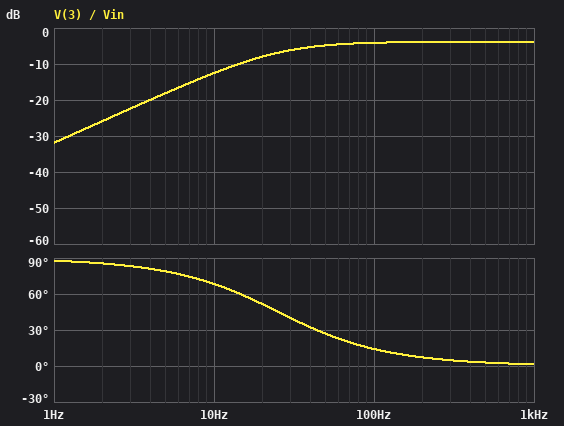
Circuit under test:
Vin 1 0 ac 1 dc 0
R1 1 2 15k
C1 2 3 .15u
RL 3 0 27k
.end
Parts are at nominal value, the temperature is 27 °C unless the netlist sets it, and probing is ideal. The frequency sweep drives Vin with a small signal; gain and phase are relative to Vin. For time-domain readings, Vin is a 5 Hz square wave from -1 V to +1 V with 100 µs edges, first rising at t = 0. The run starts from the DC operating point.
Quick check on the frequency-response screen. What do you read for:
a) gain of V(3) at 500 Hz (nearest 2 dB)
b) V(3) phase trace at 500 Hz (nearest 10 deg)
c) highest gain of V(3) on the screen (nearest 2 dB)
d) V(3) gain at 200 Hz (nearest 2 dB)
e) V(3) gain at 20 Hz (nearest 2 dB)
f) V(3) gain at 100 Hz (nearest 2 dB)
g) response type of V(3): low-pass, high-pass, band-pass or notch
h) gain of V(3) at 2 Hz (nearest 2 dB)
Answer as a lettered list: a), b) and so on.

a) -4 dB
b) 0 deg
c) -4 dB
d) -4 dB
e) -8 dB
f) -4 dB
g) high-pass
h) -26 dB
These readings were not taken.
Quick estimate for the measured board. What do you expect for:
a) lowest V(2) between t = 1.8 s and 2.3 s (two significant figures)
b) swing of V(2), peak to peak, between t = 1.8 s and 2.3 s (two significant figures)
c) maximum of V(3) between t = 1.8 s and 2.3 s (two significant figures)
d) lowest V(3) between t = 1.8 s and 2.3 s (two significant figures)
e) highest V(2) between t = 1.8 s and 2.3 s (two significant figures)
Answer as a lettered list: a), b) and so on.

a) -1.0 V
b) 2.0 V
c) 1.3 V
d) -1.3 V
e) 1.0 V
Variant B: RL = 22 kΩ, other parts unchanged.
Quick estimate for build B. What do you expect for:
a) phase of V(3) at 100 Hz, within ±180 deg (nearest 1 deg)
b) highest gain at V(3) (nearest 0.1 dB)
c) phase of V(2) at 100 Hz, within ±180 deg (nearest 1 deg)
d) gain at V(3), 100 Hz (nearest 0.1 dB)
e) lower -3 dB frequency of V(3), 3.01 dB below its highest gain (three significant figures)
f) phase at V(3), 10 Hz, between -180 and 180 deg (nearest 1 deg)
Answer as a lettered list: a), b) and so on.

a) 16 deg
b) -4.5 dB
c) -10 deg
d) -4.9 dB
e) 28.7 Hz
f) 71 deg
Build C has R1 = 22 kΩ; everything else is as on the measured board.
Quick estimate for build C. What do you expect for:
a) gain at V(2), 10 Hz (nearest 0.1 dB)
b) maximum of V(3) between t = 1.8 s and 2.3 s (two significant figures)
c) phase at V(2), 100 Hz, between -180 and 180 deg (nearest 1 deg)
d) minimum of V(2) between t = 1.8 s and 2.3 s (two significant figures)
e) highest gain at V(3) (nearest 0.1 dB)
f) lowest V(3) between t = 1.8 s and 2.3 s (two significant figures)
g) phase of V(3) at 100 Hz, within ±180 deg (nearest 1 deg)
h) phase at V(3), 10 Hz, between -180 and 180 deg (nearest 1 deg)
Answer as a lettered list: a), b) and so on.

a) -0.6 dB
b) 1.1 V
c) -9 deg
d) -1.0 V
e) -5.2 dB
f) -1.1 V
g) 12 deg
h) 65 deg
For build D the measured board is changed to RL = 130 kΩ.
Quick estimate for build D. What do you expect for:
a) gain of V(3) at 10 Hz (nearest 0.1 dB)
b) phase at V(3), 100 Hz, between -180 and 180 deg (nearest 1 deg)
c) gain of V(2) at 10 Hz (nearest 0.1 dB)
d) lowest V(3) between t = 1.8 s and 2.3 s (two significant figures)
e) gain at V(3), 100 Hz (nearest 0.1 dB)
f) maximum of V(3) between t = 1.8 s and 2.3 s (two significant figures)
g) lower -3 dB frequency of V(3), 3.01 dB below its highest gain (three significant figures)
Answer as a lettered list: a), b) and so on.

a) -2.8 dB
b) 4 deg
c) -0.6 dB
d) -1.8 V
e) -1.0 dB
f) 1.8 V
g) 7.32 Hz
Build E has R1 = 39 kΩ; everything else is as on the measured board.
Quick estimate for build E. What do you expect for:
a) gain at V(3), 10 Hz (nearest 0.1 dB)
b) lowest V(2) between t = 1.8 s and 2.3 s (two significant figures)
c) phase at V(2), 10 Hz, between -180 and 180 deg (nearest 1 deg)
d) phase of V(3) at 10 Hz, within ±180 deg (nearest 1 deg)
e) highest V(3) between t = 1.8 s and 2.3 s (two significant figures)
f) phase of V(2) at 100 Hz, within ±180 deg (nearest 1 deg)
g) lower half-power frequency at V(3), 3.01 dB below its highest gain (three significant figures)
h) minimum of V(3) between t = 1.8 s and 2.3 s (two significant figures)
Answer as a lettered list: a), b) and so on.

a) -13.3 dB
b) -1.0 V
c) -18 deg
d) 58 deg
e) 810 mV
f) -12 deg
g) 16.1 Hz
h) -810 mV
